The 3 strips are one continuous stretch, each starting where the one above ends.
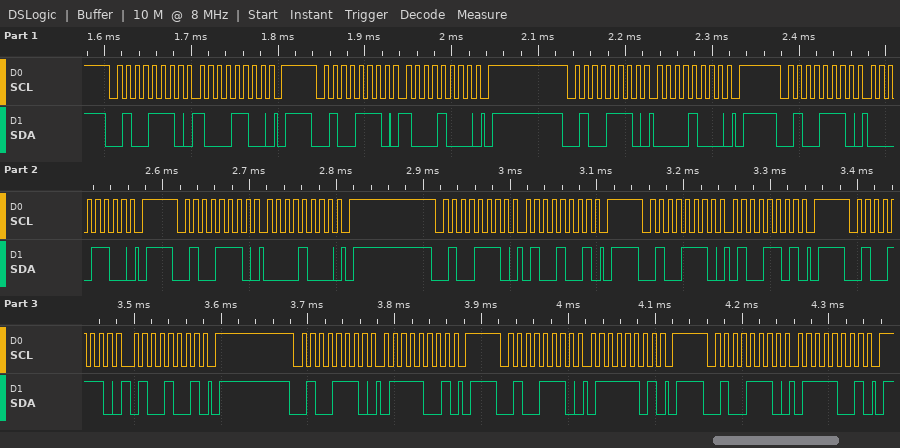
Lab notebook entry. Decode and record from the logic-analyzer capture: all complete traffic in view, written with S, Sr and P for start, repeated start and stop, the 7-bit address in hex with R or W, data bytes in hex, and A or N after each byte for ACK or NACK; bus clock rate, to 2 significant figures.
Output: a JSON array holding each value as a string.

["S 27W A 8C A P S 27W A 88 A P S 27W A 08 A P S 27W A 0C A P S 27W A 08 A P S 27W A 49 A P S 27W A 4D A P S 27W A 49 A P S 27W A 79 A P S 27W A 7D A P S 27W A 79 A P", "100 kHz"]
